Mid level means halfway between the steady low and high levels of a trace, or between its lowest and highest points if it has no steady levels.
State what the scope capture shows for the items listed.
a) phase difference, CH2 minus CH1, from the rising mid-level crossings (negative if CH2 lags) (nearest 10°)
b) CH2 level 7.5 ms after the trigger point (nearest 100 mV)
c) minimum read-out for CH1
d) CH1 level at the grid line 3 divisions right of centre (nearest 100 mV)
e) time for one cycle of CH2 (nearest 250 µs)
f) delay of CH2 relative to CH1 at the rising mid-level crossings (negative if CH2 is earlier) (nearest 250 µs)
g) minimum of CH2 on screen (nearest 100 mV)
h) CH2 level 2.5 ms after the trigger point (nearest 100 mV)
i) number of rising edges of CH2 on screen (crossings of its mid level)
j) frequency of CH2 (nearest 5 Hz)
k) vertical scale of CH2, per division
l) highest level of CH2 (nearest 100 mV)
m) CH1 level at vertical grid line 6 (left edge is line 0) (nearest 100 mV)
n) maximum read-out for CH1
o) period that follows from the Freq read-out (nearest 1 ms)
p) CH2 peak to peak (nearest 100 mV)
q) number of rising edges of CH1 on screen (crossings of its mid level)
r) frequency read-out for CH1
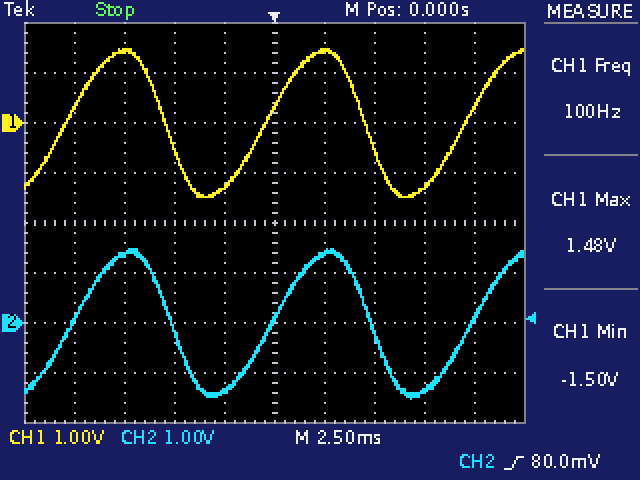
-10°
-1.3 V
-1.50 V
-1.3 V
10.00 ms
+250 µs
-1.5 V
1.4 V
3
100 Hz
1 V
1.5 V
1.4 V
1.48 V
10 ms
3.0 V
3
100 Hz
